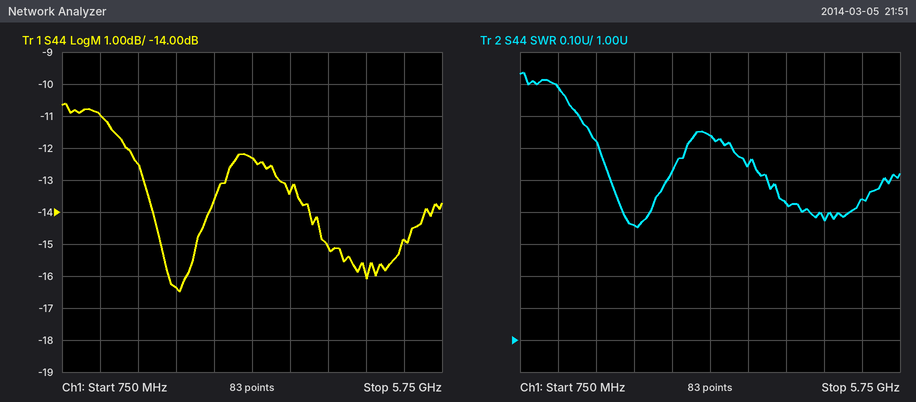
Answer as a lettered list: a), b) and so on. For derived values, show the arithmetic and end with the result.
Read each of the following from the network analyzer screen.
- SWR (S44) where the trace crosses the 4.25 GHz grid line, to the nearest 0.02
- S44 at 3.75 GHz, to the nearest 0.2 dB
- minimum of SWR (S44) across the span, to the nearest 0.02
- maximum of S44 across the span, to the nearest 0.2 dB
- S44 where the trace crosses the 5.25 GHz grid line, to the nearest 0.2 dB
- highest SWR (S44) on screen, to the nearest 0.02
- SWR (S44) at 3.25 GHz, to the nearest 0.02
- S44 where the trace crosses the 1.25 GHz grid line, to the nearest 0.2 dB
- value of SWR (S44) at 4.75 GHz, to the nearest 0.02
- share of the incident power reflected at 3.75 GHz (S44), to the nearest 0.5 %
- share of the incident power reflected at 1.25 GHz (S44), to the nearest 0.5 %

a) 1.42
b) -13.4 dB
c) 1.36
d) -10.6 dB
e) -14.8 dB
f) 1.84
g) 1.64
h) -11.0 dB
i) 1.38
j) 10^(-13.4/10) ≈ 4.57 %, so 4.5 % to the nearest 0.5 %
k) 10^(-11/10) ≈ 7.94 %, so 8.0 % to the nearest 0.5 %
